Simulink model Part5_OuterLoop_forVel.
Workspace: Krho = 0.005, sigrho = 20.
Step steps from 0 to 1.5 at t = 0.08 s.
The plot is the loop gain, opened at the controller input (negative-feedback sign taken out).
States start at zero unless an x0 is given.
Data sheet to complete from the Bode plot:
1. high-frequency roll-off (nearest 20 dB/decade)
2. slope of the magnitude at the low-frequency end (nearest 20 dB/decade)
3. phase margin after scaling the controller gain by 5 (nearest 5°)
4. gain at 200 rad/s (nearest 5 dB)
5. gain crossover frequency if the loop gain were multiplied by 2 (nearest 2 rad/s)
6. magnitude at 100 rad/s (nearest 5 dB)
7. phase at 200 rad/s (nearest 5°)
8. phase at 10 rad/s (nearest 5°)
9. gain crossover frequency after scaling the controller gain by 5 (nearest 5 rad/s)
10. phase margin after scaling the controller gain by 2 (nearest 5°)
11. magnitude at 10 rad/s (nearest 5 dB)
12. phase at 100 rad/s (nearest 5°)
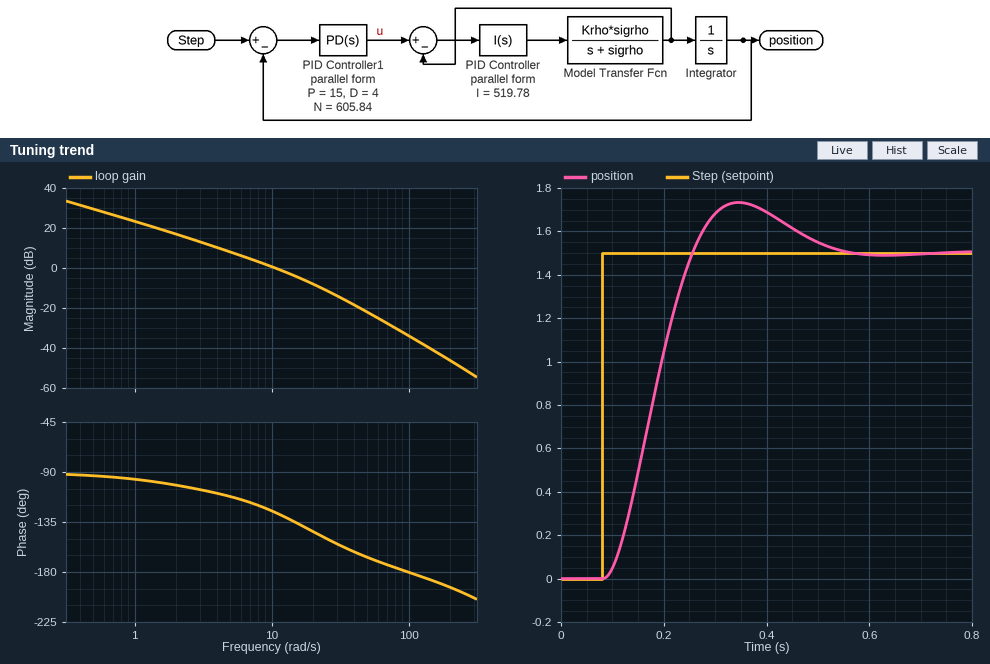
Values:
-40 dB/decade
-20 dB/decade
25°
-45 dB
18 rad/s
-35 dB
-195°
-125°
30 rad/s
40°
0 dB
-180°
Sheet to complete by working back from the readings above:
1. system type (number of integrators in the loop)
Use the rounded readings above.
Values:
1
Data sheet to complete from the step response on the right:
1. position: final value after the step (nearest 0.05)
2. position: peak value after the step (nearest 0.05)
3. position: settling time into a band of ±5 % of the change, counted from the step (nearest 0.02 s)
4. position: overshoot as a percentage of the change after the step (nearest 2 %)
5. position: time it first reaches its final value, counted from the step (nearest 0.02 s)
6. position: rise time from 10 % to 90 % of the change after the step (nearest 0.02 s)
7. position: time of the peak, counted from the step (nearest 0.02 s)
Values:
1.50
1.75
0.40 s
16 %
0.18 s
0.12 s
0.26 s
